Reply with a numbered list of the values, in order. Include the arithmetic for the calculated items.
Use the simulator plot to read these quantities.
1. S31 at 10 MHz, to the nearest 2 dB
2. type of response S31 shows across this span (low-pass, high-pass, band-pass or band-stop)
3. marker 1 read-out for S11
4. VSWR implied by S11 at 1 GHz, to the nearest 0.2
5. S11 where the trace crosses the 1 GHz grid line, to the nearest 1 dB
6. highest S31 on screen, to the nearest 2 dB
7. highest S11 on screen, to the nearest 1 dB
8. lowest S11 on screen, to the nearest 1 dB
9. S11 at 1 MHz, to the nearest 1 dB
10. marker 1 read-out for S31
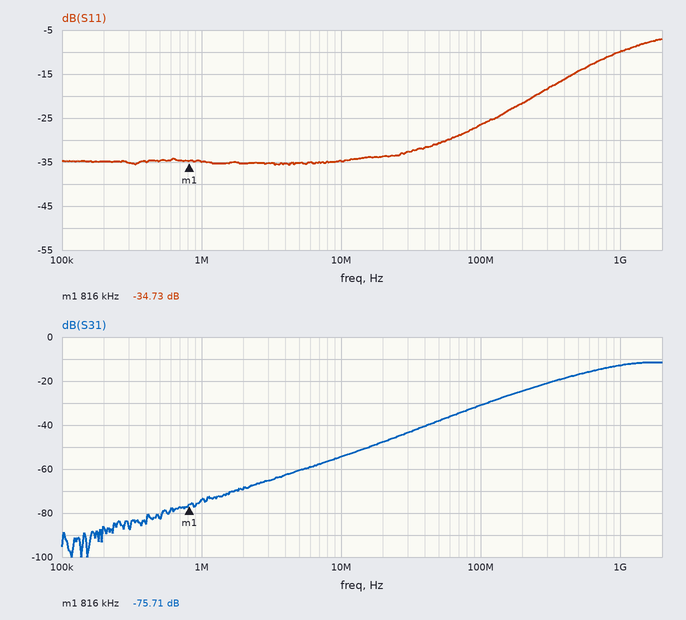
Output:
1. -54 dB
2. high-pass
3. -34.73 dB
4. |Γ| = 10^(-10/20) = 0.3162; VSWR = (1 + 0.3162)/(1 − 0.3162) ≈ 1.92, so 2.0 to the nearest 0.2
5. -10 dB
6. -12 dB
7. -7 dB
8. -36 dB
9. -35 dB
10. -75.71 dB
